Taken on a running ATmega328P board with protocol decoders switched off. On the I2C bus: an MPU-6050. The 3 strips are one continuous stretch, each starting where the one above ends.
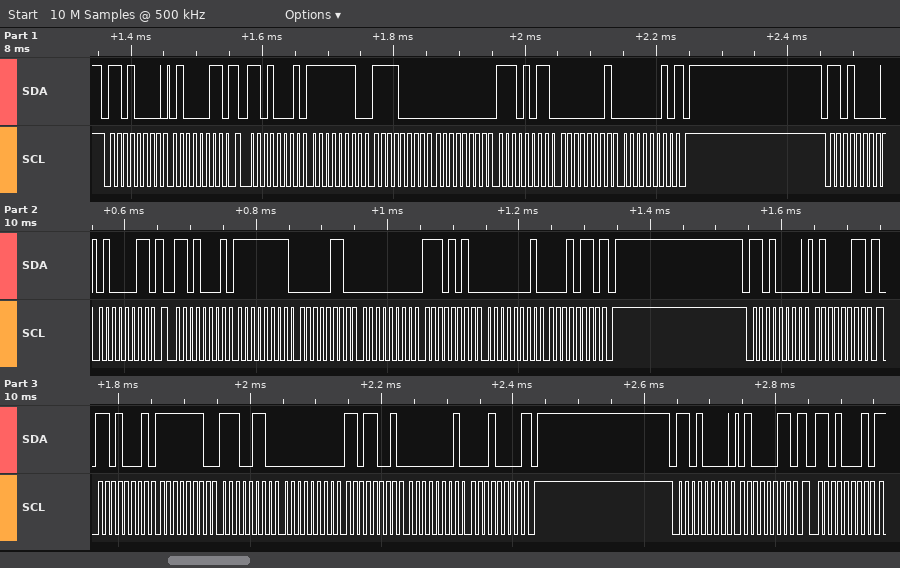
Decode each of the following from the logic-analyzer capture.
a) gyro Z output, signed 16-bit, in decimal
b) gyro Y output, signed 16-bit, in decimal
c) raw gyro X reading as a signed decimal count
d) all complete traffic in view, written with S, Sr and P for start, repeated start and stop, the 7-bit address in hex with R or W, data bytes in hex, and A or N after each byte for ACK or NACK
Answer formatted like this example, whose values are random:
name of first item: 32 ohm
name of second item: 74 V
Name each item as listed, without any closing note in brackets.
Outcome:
gyro Z output, signed 16-bit, in decimal: 258
gyro Y output, signed 16-bit, in decimal: 235
raw gyro X reading as a signed decimal count: -272
all complete traffic in view, written with S, Sr and P for start, repeated start and stop, the 7-bit address in hex with R or W, data bytes in hex, and A or N after each byte for ACK or NACK: S 68W A 43 A Sr 68R A FE A F0 A 00 A EB A 01 A 02 N P S 68W A 43 A Sr 68R A FF A 06 A 00 A EA A 01 A 16 N P S 68W A 43 A Sr 68R A FE A E6 A 00 A D9 A 01 A 10 N P S 68W A 43 A Sr 68R A
